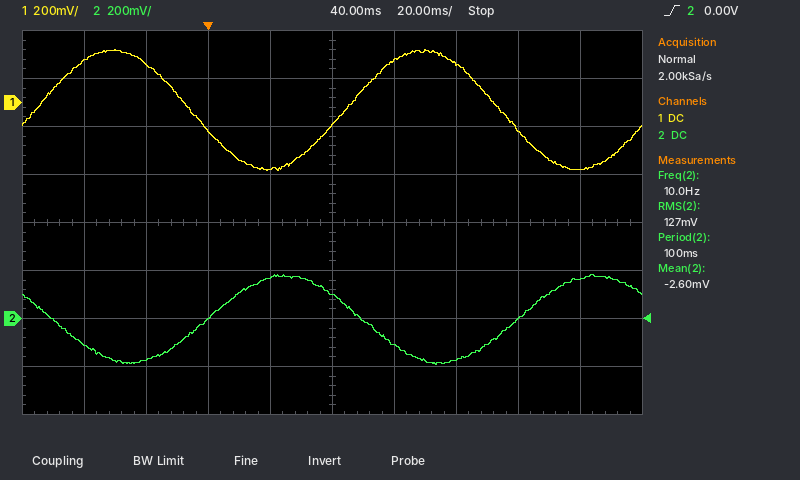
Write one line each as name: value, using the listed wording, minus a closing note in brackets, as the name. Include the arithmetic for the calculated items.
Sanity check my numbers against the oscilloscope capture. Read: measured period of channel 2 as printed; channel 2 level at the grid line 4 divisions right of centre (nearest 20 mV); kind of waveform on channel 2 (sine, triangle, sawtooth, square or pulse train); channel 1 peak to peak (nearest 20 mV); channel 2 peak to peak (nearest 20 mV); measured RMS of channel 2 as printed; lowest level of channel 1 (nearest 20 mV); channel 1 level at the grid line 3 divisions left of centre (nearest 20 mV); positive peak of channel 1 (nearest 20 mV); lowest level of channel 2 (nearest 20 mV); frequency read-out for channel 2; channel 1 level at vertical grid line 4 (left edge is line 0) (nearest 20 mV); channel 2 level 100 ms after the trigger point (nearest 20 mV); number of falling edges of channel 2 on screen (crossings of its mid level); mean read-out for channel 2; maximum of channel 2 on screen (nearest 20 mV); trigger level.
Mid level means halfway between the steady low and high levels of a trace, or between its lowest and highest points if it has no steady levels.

measured period of channel 2 as printed: 100 ms
channel 2 level at the grid line 4 divisions right of centre: 160 mV
kind of waveform on channel 2: sine
channel 1 peak to peak: 220 mV − (-280 mV) = 500 mV
channel 2 peak to peak: 180 mV − (-200 mV) = 380 mV
measured RMS of channel 2 as printed: 127 mV
lowest level of channel 1: -280 mV
channel 1 level at the grid line 3 divisions left of centre: 160 mV
positive peak of channel 1: 220 mV
lowest level of channel 2: -200 mV
frequency read-out for channel 2: 10.0 Hz
channel 1 level at vertical grid line 4 (left edge is line 0): -280 mV
channel 2 level 100 ms after the trigger point: 0 mV
number of falling edges of channel 2 on screen: 2
mean read-out for channel 2: -2.60 mV
maximum of channel 2 on screen: 180 mV
trigger level: 0.00 V
